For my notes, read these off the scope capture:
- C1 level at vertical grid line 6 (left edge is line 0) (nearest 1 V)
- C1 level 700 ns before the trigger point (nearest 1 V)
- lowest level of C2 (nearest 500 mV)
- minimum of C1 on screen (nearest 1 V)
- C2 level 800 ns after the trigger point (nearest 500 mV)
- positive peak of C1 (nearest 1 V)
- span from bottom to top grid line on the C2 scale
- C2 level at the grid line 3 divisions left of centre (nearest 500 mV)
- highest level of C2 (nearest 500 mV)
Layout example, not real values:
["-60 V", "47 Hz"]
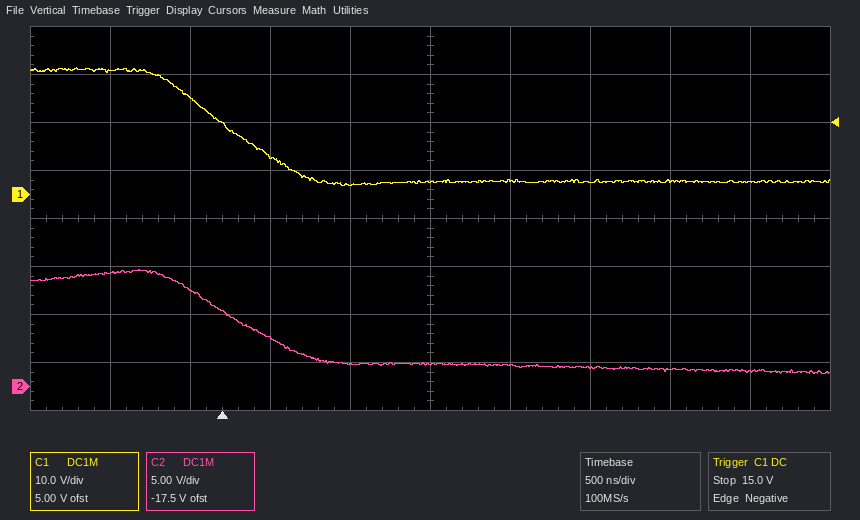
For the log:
["3 V", "26 V", "1.5 V", "2 V", "2.5 V", "26 V", "40 V", "10.0 V", "12.0 V"]
